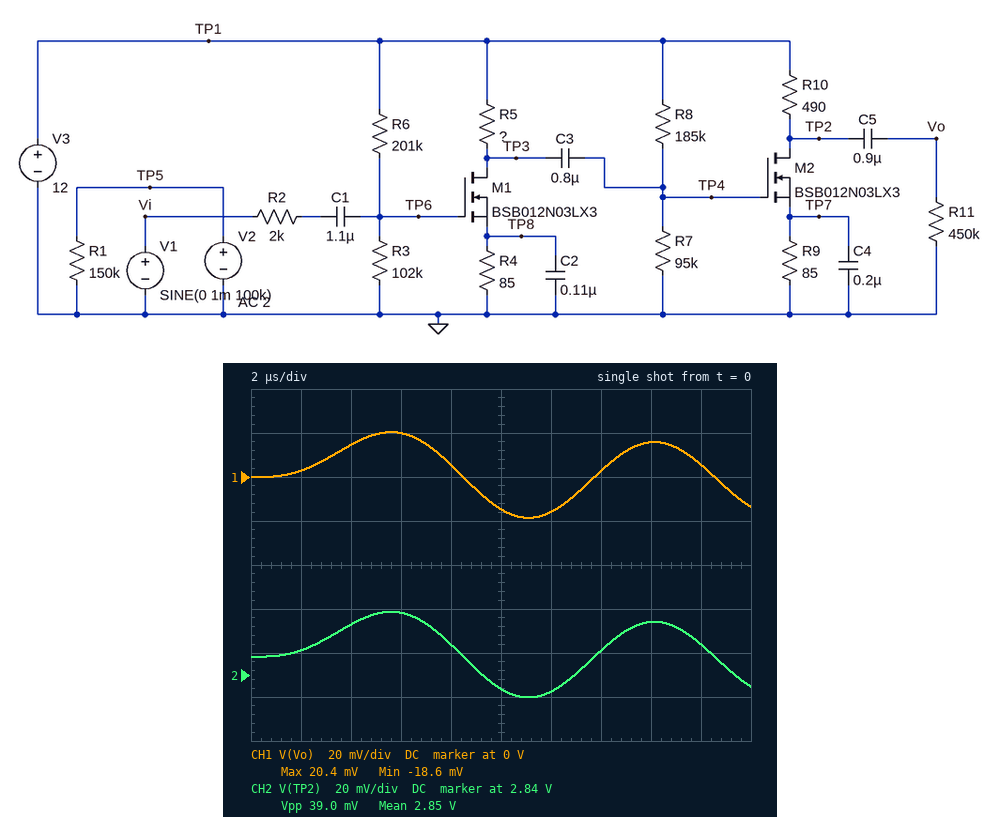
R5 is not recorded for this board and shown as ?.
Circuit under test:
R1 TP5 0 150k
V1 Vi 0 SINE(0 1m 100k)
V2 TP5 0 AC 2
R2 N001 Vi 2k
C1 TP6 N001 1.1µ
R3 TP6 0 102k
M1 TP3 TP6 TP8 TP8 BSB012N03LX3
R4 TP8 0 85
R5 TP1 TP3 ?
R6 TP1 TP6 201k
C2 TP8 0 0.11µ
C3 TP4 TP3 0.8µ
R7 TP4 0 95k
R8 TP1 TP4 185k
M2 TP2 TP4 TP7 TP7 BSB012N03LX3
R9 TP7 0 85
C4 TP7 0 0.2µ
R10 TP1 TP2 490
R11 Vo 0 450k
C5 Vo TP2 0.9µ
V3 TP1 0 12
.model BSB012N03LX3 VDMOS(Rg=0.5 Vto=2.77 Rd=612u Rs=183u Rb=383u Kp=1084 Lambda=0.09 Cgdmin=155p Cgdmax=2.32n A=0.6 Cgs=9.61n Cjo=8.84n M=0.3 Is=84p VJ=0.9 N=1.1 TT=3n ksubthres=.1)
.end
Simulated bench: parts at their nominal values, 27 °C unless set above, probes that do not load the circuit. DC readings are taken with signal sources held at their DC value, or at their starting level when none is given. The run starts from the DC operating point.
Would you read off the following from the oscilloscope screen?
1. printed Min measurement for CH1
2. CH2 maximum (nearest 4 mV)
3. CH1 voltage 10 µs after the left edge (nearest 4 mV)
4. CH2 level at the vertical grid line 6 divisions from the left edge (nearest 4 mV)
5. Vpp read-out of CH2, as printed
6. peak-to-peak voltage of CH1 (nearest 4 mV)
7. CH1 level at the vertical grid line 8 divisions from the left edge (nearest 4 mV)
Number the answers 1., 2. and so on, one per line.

1. -18.6 mV
2. 2.868 V
3. -16 mV
4. 2.832 V
5. 39.0 mV
6. 40 mV
7. 16 mV
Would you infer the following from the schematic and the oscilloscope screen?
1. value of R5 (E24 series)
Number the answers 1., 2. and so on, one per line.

1. 300 Ω
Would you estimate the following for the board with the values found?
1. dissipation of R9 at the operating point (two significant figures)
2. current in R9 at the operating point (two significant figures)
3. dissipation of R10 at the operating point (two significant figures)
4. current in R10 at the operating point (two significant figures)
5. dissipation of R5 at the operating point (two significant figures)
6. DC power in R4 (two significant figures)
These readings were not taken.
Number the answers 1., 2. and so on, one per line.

1. 30 mW
2. 19 mA
3. 170 mW
4. 19 mA
5. 100 mW
6. 29 mW
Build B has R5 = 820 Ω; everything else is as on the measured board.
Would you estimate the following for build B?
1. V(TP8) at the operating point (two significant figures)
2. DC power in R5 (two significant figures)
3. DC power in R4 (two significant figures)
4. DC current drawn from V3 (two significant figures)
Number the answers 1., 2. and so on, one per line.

1. 1.1 V
2. 140 mW
3. 15 mW
4. 32 mA
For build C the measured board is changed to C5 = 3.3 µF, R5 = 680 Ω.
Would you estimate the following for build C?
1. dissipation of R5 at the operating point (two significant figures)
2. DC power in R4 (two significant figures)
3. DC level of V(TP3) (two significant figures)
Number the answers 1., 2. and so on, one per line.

1. 170 mW
2. 21 mW
3. 1.3 V
